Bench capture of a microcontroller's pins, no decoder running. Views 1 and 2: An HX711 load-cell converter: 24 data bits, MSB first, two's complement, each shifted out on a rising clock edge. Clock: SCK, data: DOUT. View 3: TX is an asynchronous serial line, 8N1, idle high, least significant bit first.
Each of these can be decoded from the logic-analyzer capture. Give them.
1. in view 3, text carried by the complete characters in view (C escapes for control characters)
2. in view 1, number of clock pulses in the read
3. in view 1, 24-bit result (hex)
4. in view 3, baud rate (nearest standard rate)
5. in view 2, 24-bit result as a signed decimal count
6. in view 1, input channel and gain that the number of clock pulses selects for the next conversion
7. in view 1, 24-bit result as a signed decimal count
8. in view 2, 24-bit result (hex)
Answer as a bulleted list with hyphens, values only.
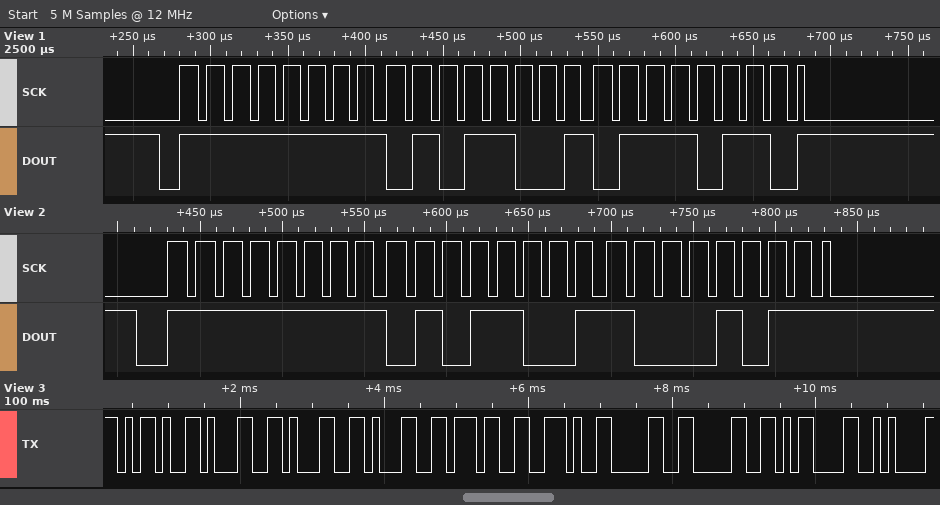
- "-1117.00\r\n"
- 25
- 0xFF5976
- 9600 baud
- -42613
- channel A, gain 128
- -42634
- 0xFF598B
